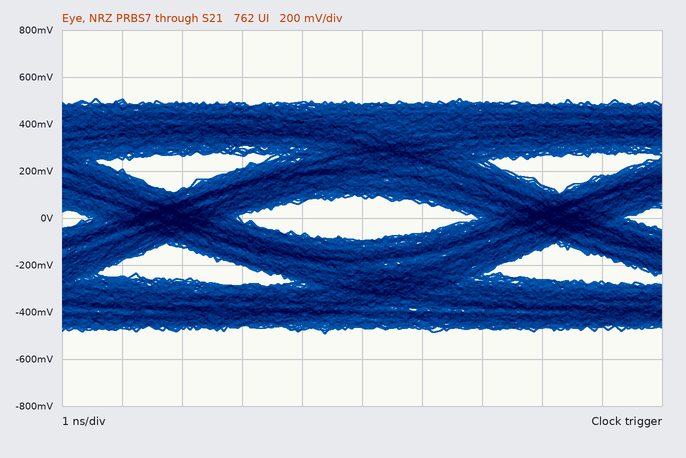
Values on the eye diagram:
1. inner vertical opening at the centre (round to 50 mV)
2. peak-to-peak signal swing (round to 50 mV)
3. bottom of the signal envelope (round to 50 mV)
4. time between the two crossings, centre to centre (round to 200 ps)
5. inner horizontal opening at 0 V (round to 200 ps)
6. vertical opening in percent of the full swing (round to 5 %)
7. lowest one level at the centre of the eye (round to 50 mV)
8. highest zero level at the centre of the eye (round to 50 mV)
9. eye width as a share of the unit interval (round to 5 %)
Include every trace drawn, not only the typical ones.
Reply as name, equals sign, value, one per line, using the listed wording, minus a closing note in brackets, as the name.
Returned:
inner vertical opening at the centre = 200 mV
peak-to-peak signal swing = 1.00 V
bottom of the signal envelope = -500 mV
time between the two crossings, centre to centre = 6.4 ns
inner horizontal opening at 0 V = 4.0 ns
vertical opening in percent of the full swing = 20 %
lowest one level at the centre of the eye = 100 mV
highest zero level at the centre of the eye = -100 mV
eye width as a share of the unit interval = 60 %
